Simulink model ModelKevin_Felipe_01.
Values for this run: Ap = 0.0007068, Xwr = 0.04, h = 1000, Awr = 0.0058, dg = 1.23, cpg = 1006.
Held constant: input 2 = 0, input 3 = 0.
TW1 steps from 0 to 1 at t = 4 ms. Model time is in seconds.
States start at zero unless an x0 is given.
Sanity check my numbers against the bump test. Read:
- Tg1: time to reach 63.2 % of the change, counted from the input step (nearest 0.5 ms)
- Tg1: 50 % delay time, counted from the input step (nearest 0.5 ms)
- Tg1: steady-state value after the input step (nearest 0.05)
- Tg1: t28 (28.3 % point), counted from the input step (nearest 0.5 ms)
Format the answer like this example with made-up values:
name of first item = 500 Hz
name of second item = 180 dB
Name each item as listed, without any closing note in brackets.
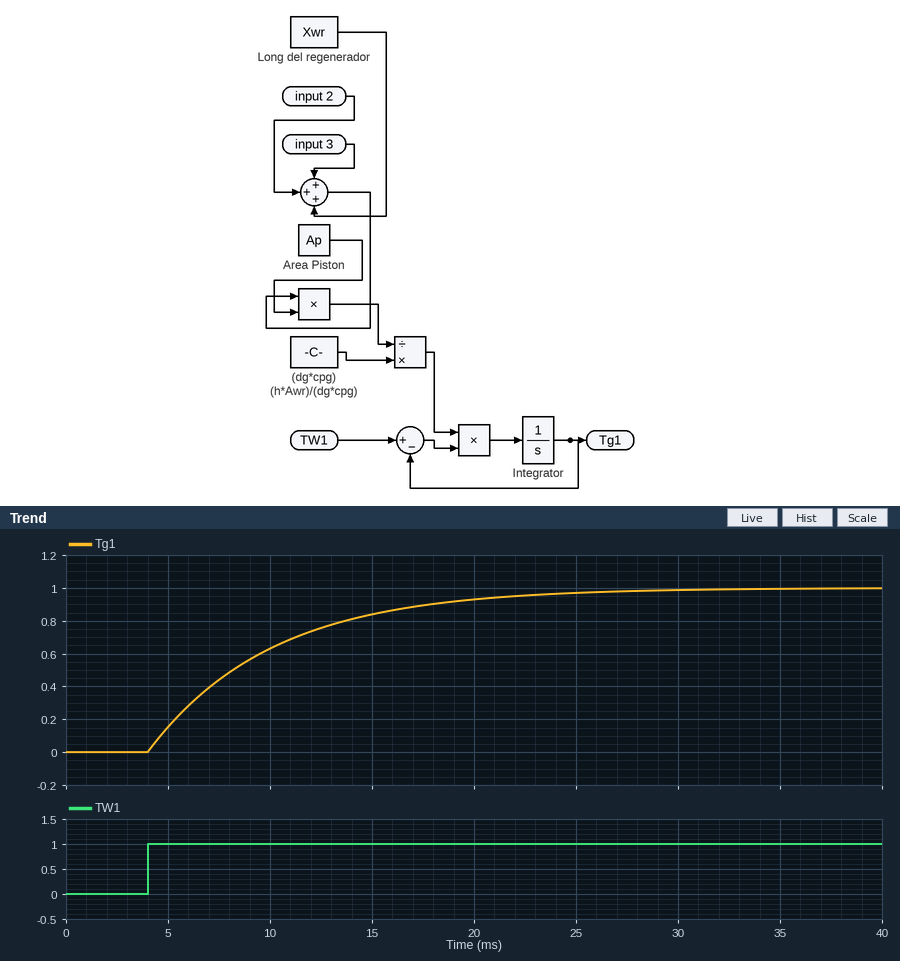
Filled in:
Tg1: time to reach 63.2 % of the change, counted from the input step = 6.0 ms
Tg1: 50 % delay time, counted from the input step = 4.0 ms
Tg1: steady-state value after the input step = 1.00
Tg1: t28 (28.3 % point), counted from the input step = 2.0 ms
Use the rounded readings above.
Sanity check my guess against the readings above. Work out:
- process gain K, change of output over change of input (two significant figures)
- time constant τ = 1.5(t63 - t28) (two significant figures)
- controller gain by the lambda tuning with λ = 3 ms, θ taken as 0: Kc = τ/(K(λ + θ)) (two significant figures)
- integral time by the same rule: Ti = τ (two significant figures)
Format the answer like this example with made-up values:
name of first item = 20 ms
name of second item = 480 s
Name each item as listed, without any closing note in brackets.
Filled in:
process gain K, change of output over change of input = 1.0
time constant τ = 1.5(t63 - t28) = 6.0 ms
controller gain by the lambda tuning with λ = 3 ms, θ taken as 0: Kc = τ/(K(λ + θ)) = 2.0
integral time by the same rule: Ti = τ = 6.0 ms
